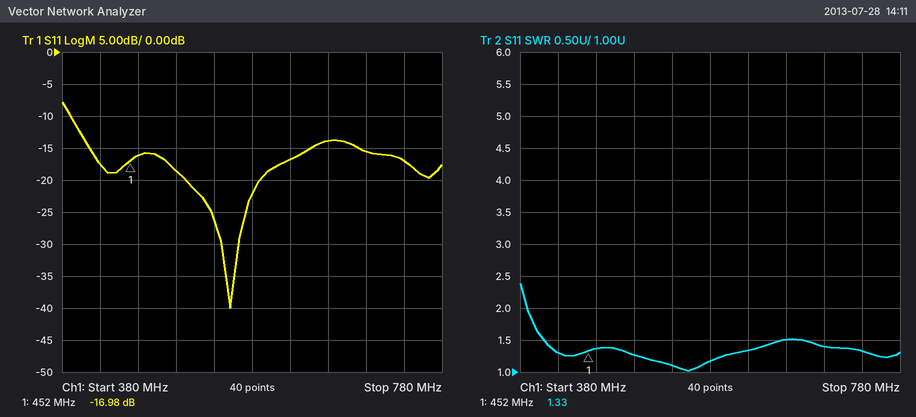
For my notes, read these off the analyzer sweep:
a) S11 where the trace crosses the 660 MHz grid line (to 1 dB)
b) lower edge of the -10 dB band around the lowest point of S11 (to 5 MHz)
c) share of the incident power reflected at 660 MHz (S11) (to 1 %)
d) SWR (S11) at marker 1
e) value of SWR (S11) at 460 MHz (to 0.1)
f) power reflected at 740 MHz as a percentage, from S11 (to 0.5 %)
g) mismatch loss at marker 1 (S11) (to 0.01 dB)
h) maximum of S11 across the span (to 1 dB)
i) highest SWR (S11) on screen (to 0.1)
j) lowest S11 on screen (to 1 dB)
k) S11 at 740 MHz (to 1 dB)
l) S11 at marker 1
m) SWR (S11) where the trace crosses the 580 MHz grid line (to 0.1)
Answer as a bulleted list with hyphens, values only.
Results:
- -14 dB
- 390 MHz
- 4 %
- 1.33
- 1.4
- 2.0 %
- 0.09 dB
- -8 dB
- 2.4
- -40 dB
- -17 dB
- -16.98 dB
- 1.2
